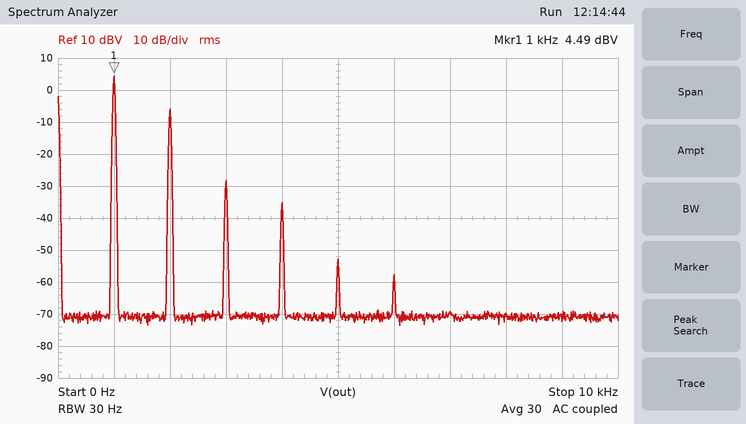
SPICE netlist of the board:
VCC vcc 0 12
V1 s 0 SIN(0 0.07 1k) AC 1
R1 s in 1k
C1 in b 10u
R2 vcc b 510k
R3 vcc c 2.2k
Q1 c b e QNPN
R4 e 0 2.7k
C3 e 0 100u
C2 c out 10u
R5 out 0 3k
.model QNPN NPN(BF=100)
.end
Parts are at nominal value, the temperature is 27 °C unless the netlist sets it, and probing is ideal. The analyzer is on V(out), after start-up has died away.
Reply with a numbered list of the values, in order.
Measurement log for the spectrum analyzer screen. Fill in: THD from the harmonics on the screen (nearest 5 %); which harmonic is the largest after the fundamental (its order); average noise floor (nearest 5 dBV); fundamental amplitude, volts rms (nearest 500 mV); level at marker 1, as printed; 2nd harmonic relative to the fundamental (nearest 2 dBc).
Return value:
1. 30 %
2. 2
3. -70 dBV
4. 1.5 V
5. 4.49 dBV
6. -10 dBc
